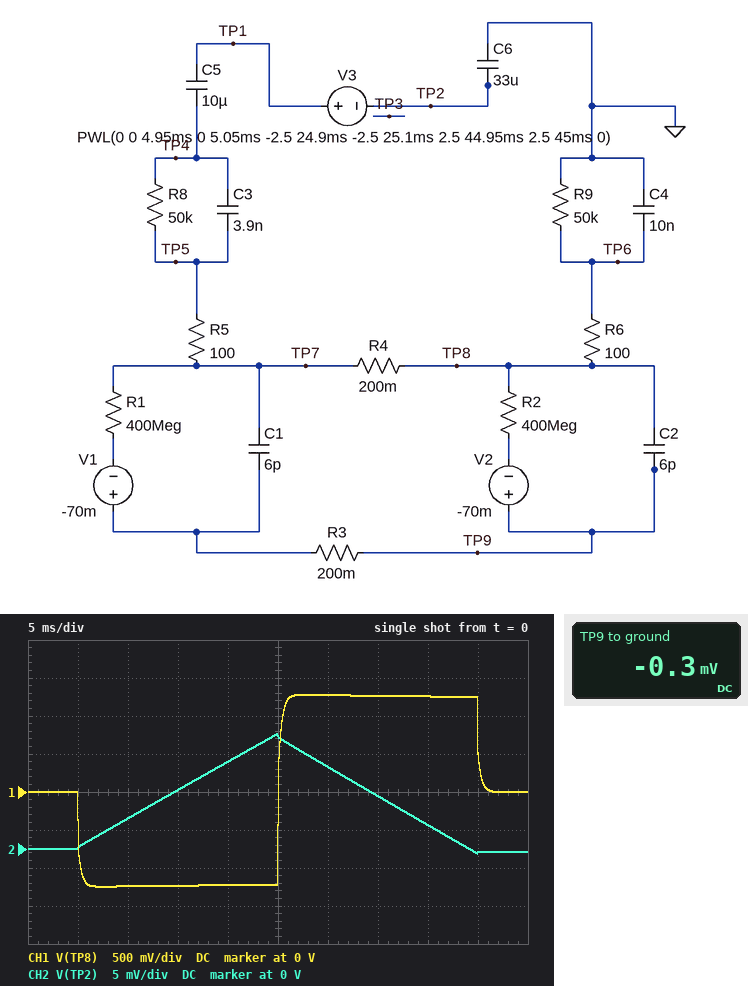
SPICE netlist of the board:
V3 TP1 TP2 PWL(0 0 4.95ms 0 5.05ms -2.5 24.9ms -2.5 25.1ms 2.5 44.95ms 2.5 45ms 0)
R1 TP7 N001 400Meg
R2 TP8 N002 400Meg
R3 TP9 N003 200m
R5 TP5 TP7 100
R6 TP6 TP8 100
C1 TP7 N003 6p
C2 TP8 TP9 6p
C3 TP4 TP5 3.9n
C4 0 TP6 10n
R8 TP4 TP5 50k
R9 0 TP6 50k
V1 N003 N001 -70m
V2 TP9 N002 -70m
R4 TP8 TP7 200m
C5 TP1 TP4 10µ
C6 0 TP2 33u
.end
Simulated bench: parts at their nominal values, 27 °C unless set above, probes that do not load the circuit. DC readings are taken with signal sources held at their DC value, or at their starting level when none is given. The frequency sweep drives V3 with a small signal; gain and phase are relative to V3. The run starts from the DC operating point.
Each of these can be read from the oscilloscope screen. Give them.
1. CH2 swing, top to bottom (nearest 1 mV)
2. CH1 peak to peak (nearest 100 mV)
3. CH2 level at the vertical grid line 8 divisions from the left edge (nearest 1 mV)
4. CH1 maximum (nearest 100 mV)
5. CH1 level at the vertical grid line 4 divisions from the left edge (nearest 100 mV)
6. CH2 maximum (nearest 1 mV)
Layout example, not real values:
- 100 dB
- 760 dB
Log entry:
- 16 mV
- 2.5 V
- 3 mV
- 1.3 V
- -1.2 V
- 15 mV
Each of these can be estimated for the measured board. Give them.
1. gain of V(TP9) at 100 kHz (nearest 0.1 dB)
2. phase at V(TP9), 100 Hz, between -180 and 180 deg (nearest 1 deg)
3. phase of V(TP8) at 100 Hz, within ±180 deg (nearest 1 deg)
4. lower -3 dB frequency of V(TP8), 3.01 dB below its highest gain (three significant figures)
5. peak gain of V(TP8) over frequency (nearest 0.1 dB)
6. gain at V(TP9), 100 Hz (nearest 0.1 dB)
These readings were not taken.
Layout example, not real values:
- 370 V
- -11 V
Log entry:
- -10.1 dB
- -5 deg
- -5 deg
- 207 mHz
- -6.0 dB
- -6.2 dB
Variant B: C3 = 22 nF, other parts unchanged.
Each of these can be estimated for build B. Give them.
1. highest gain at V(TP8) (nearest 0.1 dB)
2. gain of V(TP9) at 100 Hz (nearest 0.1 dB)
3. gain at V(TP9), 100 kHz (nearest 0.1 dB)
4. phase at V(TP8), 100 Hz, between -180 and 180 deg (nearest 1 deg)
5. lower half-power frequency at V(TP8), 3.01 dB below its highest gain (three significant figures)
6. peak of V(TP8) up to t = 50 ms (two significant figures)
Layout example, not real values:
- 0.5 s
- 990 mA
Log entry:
- -3.3 dB
- -5.3 dB
- -4.2 dB
- 8 deg
- 845 mHz
- 2.1 V
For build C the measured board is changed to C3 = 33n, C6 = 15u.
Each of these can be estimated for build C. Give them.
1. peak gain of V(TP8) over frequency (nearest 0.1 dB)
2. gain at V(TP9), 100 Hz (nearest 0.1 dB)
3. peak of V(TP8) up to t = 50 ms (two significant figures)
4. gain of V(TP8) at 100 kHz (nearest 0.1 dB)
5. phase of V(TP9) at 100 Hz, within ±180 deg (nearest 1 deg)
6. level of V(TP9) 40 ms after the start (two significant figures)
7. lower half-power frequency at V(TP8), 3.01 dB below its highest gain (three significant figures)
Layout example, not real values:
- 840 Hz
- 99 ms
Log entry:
- -2.3 dB
- -4.5 dB
- 2.5 V
- -3.7 dB
- 12 deg
- 1.2 V
- 57.2 Hz
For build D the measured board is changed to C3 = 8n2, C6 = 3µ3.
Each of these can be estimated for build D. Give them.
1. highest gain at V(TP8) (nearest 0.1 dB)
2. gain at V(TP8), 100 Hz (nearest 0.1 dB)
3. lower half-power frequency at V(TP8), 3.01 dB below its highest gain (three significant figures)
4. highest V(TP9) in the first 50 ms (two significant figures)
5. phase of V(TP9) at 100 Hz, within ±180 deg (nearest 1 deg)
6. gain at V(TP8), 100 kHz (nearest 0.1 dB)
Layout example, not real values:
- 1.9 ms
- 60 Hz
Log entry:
- -6.0 dB
- -6.1 dB
- 640 mHz
- 1.3 V
- -1 deg
- -6.7 dB
